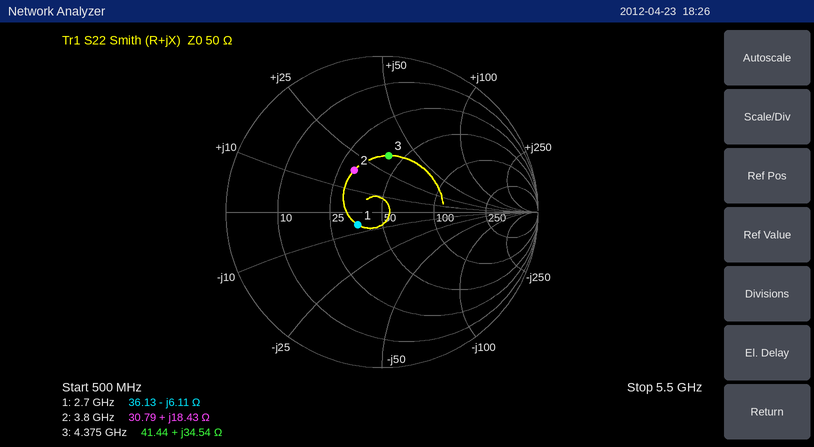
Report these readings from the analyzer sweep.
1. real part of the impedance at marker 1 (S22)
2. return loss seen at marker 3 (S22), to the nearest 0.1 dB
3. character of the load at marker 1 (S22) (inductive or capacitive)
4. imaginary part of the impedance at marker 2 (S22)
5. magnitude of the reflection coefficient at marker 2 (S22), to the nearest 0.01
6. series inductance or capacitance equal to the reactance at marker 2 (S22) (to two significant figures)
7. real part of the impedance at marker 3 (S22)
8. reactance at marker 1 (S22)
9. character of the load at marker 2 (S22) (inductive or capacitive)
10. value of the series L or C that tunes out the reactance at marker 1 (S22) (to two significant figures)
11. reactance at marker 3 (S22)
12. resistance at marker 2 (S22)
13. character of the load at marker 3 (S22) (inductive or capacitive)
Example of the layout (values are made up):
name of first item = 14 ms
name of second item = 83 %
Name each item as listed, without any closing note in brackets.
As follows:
real part of the impedance at marker 1 = 36.13 Ω
return loss seen at marker 3 (S22), to the nearest 0.1 dB = 8.8 dB
character of the load at marker 1 (S22) = capacitive
imaginary part of the impedance at marker 2 = +18.43 Ω
magnitude of the reflection coefficient at marker 2 (S22), to the nearest 0.01 = 0.32
series inductance or capacitance equal to the reactance at marker 2 (S22) = 770 pH
real part of the impedance at marker 3 = 41.44 Ω
reactance at marker 1 = -6.11 Ω
character of the load at marker 2 (S22) = inductive
value of the series L or C that tunes out the reactance at marker 1 (S22) = 360 pH
reactance at marker 3 = +34.54 Ω
resistance at marker 2 = 30.79 Ω
character of the load at marker 3 (S22) = inductive
